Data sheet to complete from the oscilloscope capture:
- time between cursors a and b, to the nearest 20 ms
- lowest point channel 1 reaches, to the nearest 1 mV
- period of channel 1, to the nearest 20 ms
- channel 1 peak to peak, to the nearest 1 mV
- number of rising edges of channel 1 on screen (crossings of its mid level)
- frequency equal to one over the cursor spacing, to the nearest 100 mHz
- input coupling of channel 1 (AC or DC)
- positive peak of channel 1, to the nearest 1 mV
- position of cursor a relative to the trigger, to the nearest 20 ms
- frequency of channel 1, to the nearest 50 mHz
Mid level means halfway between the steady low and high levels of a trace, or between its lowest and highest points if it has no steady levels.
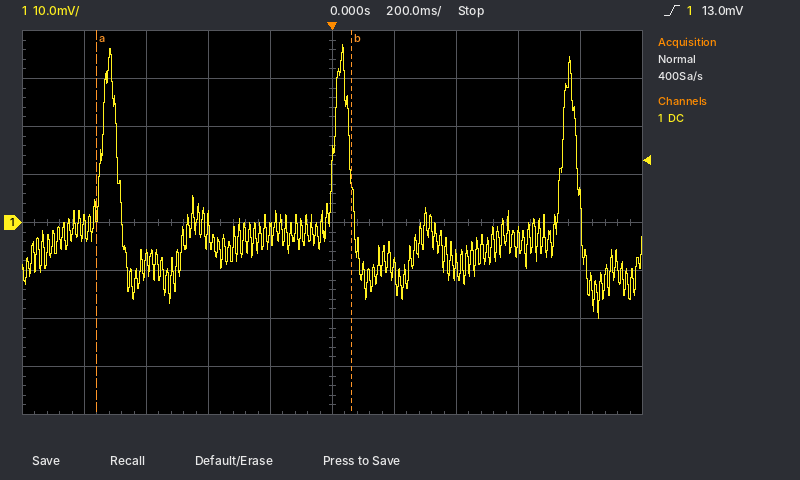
820 ms
-20 mV
740 ms
57 mV
3
1.2 Hz
DC
37 mV
-760 ms
1.35 Hz
